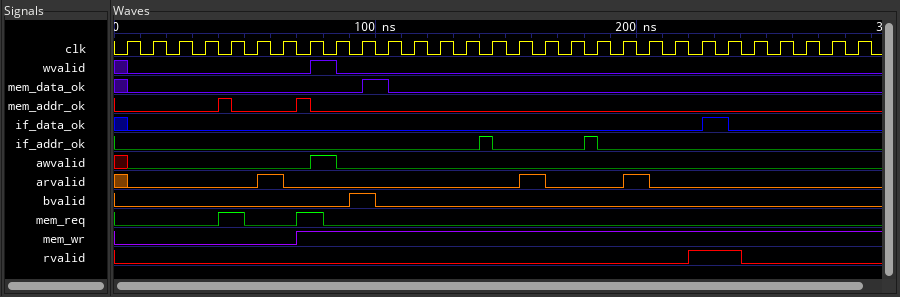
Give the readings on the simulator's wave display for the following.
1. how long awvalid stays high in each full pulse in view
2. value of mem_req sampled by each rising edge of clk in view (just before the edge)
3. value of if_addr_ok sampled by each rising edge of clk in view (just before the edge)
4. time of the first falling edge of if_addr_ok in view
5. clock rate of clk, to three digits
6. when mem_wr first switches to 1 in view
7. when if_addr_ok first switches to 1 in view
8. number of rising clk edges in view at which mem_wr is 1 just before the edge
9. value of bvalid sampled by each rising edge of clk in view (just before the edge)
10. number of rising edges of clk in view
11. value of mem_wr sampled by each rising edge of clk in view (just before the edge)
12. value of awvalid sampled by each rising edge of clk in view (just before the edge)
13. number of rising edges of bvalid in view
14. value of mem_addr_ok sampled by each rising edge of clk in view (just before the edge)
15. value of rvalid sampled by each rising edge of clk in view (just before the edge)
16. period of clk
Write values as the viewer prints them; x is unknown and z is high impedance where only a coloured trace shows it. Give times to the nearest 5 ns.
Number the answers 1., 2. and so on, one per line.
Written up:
1. 10 ns
2. 0 0 0 0 1 0 0 1 0 0 0 0 0 0 0 0 0 0 0 0 0 0 0 0 0 0 0 0 0
3. 0 0 0 0 0 0 0 0 0 0 0 0 0 0 1 0 0 0 1 0 0 0 0 0 0 0 0 0 0
4. 145 ns
5. 100 MHz
6. 70 ns
7. 140 ns
8. 22
9. 0 0 0 0 0 0 0 0 0 1 0 0 0 0 0 0 0 0 0 0 0 0 0 0 0 0 0 0 0
10. 29
11. 0 0 0 0 0 0 0 1 1 1 1 1 1 1 1 1 1 1 1 1 1 1 1 1 1 1 1 1 1
12. x 0 0 0 0 0 0 0 1 0 0 0 0 0 0 0 0 0 0 0 0 0 0 0 0 0 0 0 0
13. 1
14. 0 0 0 0 1 0 0 1 0 0 0 0 0 0 0 0 0 0 0 0 0 0 0 0 0 0 0 0 0
15. 0 0 0 0 0 0 0 0 0 0 0 0 0 0 0 0 0 0 0 0 0 0 1 1 0 0 0 0 0
16. 10 ns
